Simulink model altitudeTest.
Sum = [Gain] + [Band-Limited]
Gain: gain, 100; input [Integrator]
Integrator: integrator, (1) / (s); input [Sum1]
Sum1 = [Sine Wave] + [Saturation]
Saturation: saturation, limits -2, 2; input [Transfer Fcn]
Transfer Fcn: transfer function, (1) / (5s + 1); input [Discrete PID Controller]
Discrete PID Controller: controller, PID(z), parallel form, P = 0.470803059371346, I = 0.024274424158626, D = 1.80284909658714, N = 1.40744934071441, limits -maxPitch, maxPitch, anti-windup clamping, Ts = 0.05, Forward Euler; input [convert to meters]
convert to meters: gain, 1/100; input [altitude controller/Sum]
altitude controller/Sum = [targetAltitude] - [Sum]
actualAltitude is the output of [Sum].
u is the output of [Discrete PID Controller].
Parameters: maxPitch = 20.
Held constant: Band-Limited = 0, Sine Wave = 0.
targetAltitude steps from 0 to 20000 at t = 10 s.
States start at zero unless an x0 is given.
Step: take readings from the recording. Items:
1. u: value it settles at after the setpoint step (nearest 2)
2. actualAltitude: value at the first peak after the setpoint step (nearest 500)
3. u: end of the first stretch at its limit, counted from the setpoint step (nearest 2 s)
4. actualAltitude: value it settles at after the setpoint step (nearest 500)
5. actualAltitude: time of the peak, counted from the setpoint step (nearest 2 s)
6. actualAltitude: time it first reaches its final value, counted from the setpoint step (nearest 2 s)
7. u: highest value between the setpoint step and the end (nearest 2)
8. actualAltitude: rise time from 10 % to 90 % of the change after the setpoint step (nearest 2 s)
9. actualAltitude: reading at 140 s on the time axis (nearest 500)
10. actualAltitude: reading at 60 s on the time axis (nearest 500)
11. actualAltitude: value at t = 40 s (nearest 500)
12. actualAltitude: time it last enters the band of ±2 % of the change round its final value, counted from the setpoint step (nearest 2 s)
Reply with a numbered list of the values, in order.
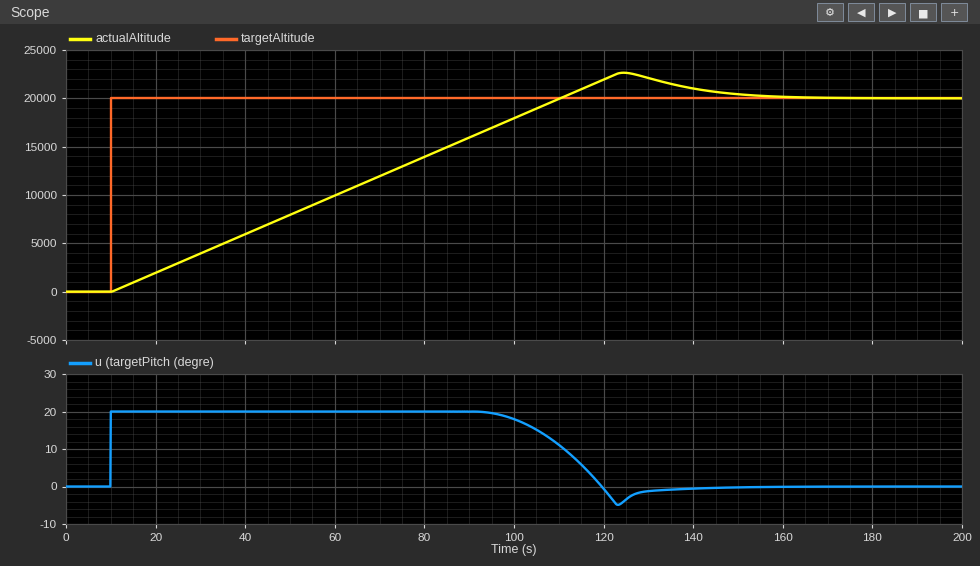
1. 0
2. 22500
3. 84 s
4. 20000
5. 114 s
6. 100 s
7. 20
8. 80 s
9. 21000
10. 10000
11. 6000
12. 140 s
